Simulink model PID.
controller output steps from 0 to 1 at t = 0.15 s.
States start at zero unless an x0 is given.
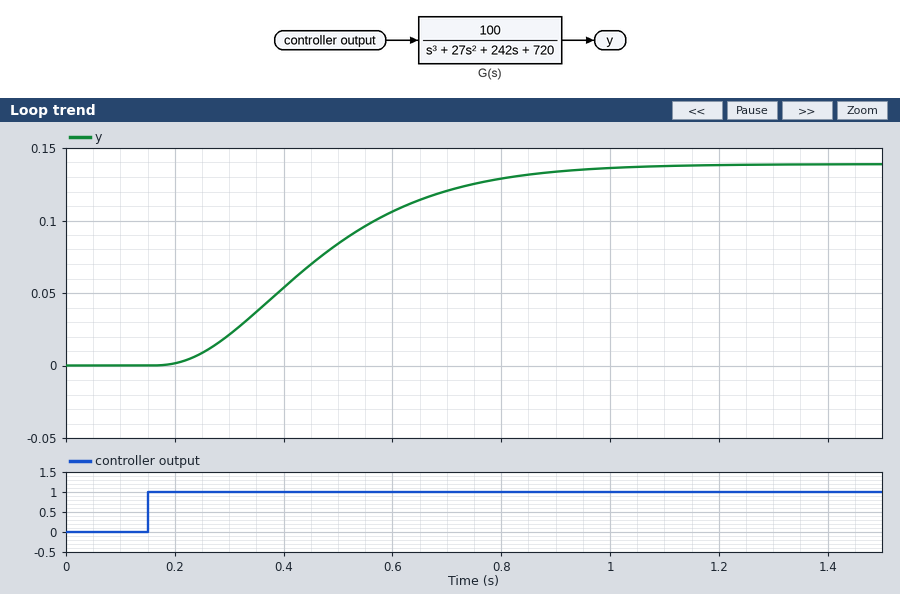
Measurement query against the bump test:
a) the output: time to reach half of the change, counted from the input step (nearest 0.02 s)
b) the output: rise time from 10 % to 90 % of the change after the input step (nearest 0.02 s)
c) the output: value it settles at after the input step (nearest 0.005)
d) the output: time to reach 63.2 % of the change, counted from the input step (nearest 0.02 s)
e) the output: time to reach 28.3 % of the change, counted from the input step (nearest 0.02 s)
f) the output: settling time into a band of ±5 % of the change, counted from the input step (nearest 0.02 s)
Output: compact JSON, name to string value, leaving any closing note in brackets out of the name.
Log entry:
{"the output: time to reach half of the change, counted from the input step": "0.30 s", "the output: rise time from 10 % to 90 % of the change after the input step": "0.48 s", "the output: value it settles at after the input step": "0.140", "the output: time to reach 63.2 % of the change, counted from the input step": "0.36 s", "the output: time to reach 28.3 % of the change, counted from the input step": "0.20 s", "the output: settling time into a band of ±5 % of the change, counted from the input step": "0.70 s"}
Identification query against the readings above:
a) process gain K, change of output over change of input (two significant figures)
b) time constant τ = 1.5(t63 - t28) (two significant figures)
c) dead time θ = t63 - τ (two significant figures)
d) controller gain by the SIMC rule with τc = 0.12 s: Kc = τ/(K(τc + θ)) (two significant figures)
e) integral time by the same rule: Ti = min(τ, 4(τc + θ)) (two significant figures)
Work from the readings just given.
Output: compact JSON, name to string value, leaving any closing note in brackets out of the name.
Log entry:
{"process gain K, change of output over change of input": "0.14", "time constant τ = 1.5(t63 - t28)": "0.24 s", "dead time θ = t63 - τ": "0.12 s", "controller gain by the SIMC rule with τc = 0.12 s: Kc = τ/(K(τc + θ))": "7.1", "integral time by the same rule: Ti = min(τ, 4(τc + θ))": "0.24 s"}
